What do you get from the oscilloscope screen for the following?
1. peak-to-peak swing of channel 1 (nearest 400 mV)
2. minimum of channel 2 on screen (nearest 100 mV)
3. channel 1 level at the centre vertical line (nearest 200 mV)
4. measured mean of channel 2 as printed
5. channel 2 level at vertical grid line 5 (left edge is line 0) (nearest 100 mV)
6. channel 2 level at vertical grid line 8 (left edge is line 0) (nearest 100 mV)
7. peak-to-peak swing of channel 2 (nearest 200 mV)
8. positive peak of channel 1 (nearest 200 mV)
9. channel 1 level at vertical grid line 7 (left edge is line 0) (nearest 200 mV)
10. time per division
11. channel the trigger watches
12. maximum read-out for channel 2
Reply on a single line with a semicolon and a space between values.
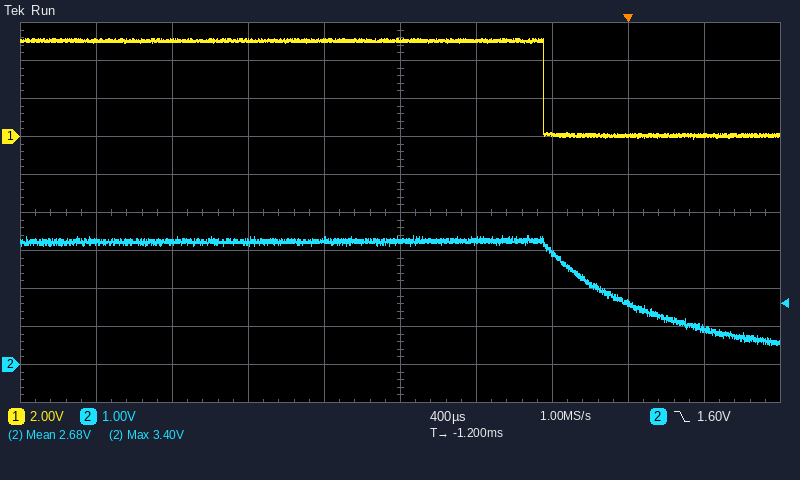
5.2 V; 500 mV; 5.0 V; 2.68 V; 3.3 V; 1.6 V; 2.8 V; 5.2 V; 200 mV; 400 µs; channel 2; 3.40 V
